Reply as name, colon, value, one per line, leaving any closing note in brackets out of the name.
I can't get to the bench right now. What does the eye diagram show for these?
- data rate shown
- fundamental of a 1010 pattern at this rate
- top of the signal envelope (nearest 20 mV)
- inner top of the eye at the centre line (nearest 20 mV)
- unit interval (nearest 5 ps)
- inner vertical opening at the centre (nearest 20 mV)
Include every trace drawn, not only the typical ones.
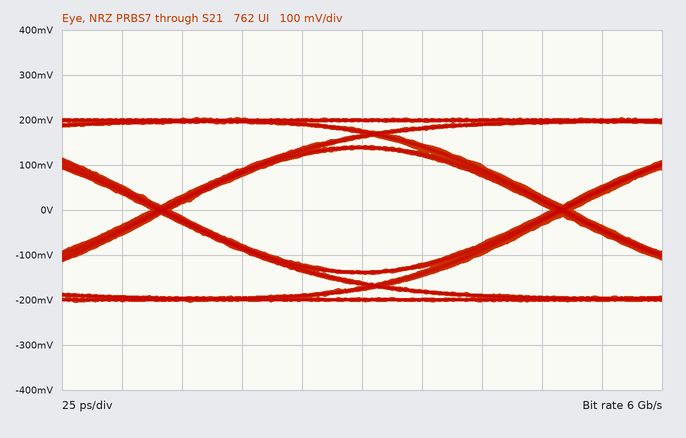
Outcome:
data rate shown: 6 Gb/s
fundamental of a 1010 pattern at this rate: 3 GHz
top of the signal envelope: 200 mV
inner top of the eye at the centre line: 140 mV
unit interval: 165 ps
inner vertical opening at the centre: 280 mV
